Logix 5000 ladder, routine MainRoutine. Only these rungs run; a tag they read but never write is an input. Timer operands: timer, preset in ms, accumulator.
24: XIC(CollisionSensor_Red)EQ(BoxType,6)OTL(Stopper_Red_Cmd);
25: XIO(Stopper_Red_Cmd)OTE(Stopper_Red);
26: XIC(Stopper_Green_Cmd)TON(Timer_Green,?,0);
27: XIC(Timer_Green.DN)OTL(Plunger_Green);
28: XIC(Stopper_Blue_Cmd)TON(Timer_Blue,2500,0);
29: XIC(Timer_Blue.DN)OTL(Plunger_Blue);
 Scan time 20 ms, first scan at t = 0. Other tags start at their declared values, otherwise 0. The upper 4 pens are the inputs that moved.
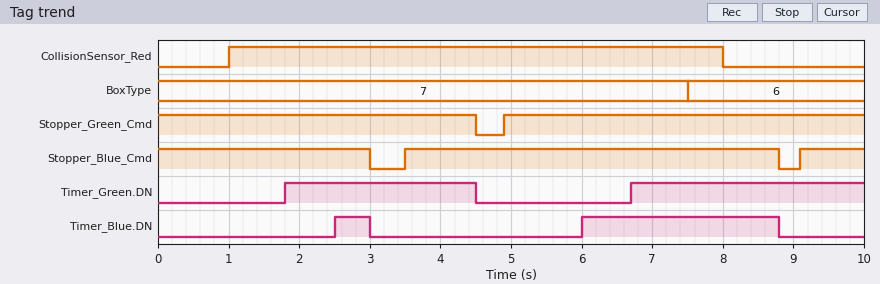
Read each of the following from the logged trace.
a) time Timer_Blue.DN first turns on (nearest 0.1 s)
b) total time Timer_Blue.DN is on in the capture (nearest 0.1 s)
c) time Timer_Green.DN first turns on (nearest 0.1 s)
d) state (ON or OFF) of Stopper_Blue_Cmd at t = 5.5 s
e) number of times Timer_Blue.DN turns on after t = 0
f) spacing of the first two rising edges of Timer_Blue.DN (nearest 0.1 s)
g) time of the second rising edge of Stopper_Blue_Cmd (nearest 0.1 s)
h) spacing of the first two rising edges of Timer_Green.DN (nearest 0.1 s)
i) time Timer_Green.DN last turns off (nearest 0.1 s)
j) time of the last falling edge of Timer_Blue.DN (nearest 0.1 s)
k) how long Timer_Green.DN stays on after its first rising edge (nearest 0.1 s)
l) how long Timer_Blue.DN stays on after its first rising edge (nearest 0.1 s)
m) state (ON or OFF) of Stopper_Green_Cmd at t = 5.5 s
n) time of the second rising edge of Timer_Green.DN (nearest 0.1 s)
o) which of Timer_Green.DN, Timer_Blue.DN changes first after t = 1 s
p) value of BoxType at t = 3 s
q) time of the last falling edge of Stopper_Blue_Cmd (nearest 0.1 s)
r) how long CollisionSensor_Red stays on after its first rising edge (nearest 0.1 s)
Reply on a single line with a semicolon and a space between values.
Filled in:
2.5 s; 3.3 s; 1.8 s; ON; 2; 3.5 s; 9.1 s; 4.9 s; 4.5 s; 8.8 s; 2.7 s; 0.5 s; ON; 6.7 s; Timer_Green.DN; 7; 8.8 s; 7.0 s
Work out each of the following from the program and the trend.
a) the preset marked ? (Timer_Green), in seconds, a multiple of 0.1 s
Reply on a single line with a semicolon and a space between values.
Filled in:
1.8 s
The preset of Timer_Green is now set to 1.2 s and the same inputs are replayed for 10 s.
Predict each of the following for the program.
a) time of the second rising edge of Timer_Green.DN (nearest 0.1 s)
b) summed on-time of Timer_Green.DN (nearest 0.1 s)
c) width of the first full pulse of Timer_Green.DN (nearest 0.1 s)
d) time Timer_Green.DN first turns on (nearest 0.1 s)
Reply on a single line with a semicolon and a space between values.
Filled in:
6.1 s; 7.2 s; 3.3 s; 1.2 s
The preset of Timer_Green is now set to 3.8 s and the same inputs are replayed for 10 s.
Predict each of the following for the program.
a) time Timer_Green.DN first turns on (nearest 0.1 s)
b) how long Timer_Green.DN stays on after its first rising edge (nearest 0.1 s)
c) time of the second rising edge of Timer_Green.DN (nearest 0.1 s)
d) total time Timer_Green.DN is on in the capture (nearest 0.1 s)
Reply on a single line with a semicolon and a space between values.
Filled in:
3.8 s; 0.7 s; 8.7 s; 2.0 s
